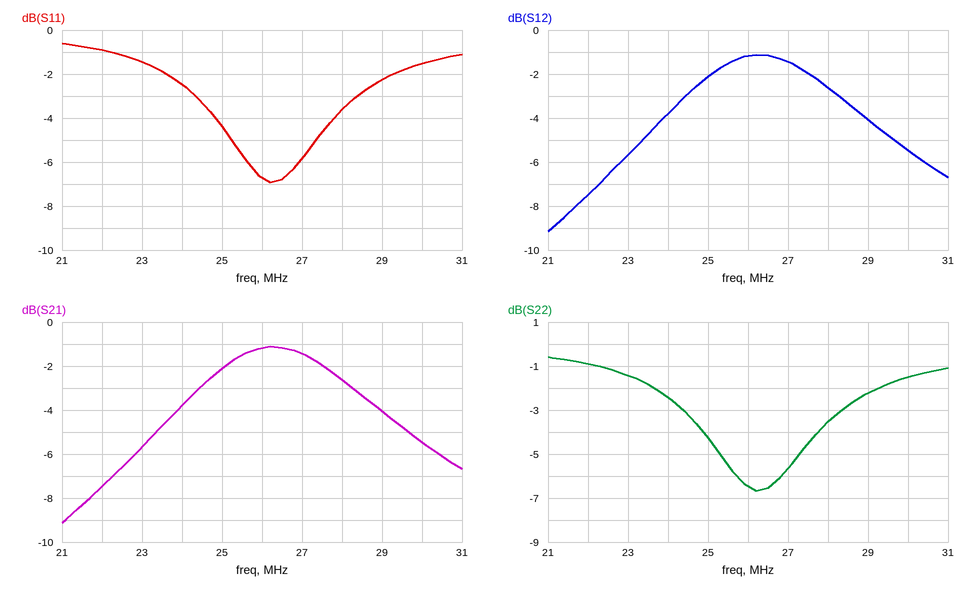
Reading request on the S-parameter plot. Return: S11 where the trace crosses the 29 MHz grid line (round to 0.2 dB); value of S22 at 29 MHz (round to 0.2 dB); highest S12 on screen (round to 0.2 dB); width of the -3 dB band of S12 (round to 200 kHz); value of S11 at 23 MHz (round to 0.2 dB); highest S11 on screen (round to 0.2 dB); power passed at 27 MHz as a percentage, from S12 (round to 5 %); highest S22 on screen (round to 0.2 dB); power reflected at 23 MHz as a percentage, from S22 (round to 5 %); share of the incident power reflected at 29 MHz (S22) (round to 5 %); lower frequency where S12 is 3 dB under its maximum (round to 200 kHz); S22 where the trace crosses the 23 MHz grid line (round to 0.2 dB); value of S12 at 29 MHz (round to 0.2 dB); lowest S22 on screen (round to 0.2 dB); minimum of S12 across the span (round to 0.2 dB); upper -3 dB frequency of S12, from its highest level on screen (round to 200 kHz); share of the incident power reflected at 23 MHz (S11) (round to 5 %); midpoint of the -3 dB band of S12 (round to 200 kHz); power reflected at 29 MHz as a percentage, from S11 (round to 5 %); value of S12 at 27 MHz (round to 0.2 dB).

-2.2 dB
-2.2 dB
-1.2 dB
5.2 MHz
-1.4 dB
-0.6 dB
70 %
-0.6 dB
70 %
60 %
23.8 MHz
-1.4 dB
-4.0 dB
-6.6 dB
-9.2 dB
29.0 MHz
70 %
26.4 MHz
60 %
-1.4 dB
